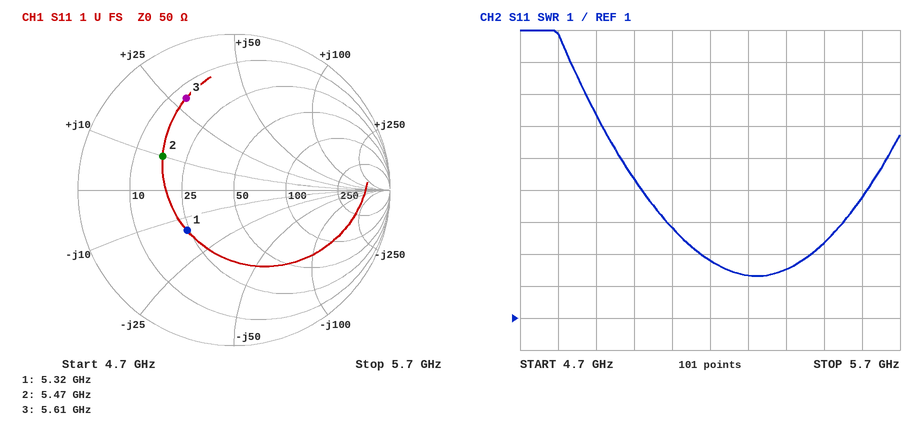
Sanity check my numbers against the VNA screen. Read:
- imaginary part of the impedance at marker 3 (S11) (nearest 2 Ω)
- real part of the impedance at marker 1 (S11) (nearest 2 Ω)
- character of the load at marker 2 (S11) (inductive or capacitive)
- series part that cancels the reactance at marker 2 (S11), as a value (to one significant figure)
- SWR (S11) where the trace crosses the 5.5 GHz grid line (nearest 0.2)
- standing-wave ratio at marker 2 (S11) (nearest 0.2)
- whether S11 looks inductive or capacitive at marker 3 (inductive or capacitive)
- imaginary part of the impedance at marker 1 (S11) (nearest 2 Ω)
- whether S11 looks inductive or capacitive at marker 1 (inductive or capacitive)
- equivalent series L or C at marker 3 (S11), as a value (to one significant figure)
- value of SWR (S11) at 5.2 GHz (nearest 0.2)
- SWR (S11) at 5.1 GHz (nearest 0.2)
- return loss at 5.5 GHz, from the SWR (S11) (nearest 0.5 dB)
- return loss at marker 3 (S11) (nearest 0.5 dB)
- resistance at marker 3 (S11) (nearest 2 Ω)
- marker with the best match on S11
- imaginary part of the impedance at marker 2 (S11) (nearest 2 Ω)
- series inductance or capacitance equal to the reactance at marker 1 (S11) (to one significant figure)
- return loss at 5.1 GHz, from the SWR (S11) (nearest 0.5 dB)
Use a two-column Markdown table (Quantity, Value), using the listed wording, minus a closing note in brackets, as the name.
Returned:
| Quantity | Value |
|---|---|
| imaginary part of the impedance at marker 3 (S11) | +28 Ω |
| real part of the impedance at marker 1 (S11) | 24 Ω |
| character of the load at marker 2 (S11) | inductive |
| series part that cancels the reactance at marker 2 (S11), as a value | 3 pF |
| SWR (S11) where the trace crosses the 5.5 GHz grid line | 3.4 |
| standing-wave ratio at marker 2 (S11) | 3.0 |
| whether S11 looks inductive or capacitive at marker 3 | inductive |
| imaginary part of the impedance at marker 1 (S11) | -14 Ω |
| whether S11 looks inductive or capacitive at marker 1 | capacitive |
| equivalent series L or C at marker 3 (S11), as a value | 800 pH |
| value of SWR (S11) at 5.2 GHz | 2.8 |
| SWR (S11) at 5.1 GHz | 3.8 |
| return loss at 5.5 GHz, from the SWR (S11) | 5.5 dB |
| return loss at marker 3 (S11) | 3.5 dB |
| resistance at marker 3 (S11) | 14 Ω |
| marker with the best match on S11 | marker 1 |
| imaginary part of the impedance at marker 2 (S11) | +10 Ω |
| series inductance or capacitance equal to the reactance at marker 1 (S11) | 2 pF |
| return loss at 5.1 GHz, from the SWR (S11) | 4.5 dB |
